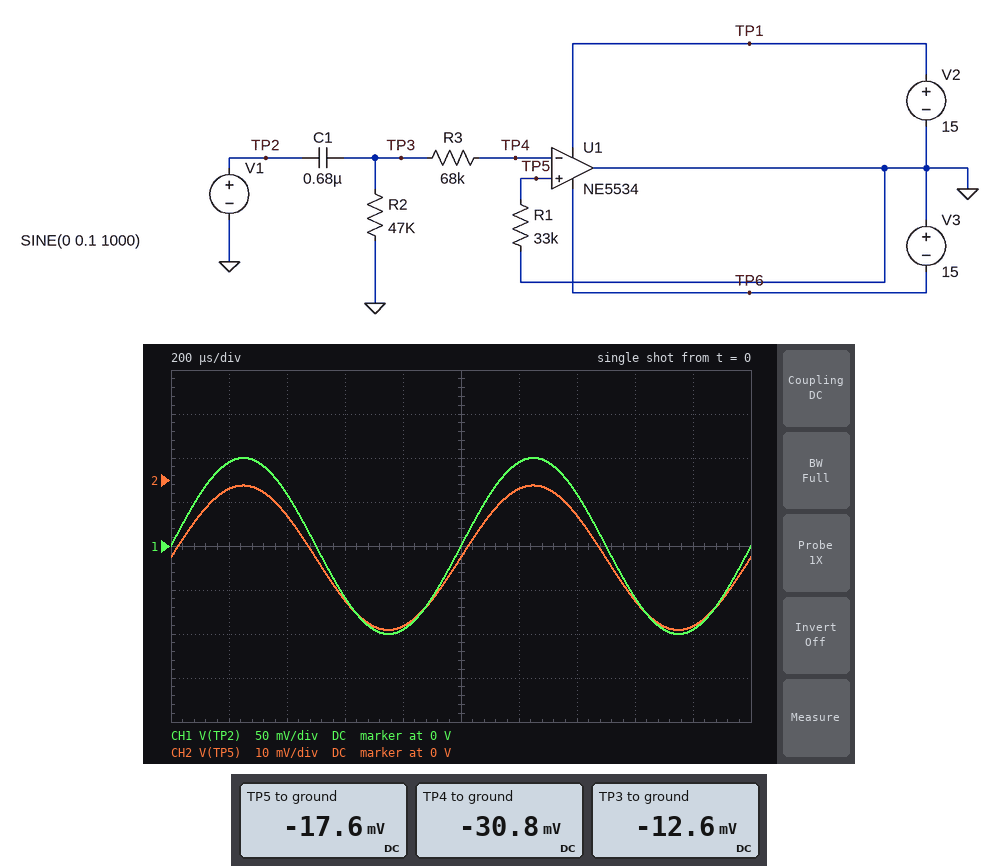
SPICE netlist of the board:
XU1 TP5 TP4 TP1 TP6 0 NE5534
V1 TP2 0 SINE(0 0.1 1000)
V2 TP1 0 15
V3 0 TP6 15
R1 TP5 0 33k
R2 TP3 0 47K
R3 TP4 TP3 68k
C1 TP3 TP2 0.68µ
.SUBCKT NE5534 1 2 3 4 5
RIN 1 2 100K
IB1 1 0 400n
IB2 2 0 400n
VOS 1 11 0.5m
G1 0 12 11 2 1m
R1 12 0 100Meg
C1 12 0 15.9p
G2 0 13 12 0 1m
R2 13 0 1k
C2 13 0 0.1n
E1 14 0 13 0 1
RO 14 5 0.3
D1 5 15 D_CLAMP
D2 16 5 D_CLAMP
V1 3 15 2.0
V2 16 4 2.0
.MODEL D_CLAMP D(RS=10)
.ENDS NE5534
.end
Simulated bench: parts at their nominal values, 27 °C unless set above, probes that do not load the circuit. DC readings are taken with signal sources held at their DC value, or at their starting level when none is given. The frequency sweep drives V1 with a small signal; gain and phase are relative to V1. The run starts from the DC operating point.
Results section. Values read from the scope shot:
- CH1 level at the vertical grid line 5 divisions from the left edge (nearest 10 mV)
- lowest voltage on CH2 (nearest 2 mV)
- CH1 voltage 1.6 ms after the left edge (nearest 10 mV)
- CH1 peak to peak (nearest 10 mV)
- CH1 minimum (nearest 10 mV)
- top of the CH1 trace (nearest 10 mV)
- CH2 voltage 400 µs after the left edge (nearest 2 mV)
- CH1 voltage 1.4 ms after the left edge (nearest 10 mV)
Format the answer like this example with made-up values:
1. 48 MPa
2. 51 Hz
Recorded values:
1. 0 V
2. -34 mV
3. -60 mV
4. 200 mV
5. -100 mV
6. 100 mV
7. -8 mV
8. 60 mV
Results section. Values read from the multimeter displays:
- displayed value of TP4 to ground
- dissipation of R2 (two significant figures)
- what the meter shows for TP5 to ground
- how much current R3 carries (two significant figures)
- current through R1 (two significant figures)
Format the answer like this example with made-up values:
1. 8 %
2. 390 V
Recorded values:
1. -30.8 mV
2. 3.4 nW
3. -17.6 mV
4. 270 nA
5. 530 nA
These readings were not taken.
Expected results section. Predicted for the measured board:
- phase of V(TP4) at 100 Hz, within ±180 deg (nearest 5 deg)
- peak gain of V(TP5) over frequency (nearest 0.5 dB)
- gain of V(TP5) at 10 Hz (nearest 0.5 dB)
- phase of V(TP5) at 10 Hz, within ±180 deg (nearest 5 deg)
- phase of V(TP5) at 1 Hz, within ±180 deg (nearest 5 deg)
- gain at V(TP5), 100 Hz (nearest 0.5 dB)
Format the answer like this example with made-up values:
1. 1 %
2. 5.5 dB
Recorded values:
1. 5 deg
2. -15.5 dB
3. -17.0 dB
4. 30 deg
5. 80 deg
6. -15.5 dB
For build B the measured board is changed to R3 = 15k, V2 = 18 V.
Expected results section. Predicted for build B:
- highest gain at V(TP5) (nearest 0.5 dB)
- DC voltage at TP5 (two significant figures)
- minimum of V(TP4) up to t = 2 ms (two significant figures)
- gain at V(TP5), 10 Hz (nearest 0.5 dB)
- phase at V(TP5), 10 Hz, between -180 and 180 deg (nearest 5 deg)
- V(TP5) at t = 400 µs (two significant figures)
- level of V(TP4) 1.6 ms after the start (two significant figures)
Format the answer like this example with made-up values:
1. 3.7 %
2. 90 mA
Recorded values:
1. -13.0 dB
2. -15 mV
3. -110 mV
4. -14.5 dB
5. 35 deg
6. -2.3 mV
7. -75 mV
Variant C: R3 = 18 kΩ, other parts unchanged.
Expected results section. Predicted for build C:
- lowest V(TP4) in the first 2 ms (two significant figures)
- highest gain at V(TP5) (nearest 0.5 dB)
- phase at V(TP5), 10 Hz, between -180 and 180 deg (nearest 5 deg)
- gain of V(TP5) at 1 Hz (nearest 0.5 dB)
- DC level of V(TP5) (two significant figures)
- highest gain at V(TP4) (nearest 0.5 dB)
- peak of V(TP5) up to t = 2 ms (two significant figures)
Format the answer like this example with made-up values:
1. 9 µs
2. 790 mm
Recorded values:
1. -110 mV
2. -13.0 dB
3. 35 deg
4. -29.5 dB
5. -15 mV
6. -1.0 dB
7. 6.4 mV
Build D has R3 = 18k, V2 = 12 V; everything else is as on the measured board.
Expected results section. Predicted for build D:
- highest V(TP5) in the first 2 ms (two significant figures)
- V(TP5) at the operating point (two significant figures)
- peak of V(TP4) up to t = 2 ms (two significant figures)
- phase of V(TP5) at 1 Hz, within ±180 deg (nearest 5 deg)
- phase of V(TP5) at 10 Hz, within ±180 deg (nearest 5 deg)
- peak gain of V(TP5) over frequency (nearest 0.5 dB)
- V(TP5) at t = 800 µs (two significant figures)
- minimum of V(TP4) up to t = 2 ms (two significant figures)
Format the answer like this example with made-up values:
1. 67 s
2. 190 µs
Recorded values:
1. 6.4 mV
2. -15 mV
3. 66 mV
4. 80 deg
5. 35 deg
6. -13.0 dB
7. -36 mV
8. -110 mV
